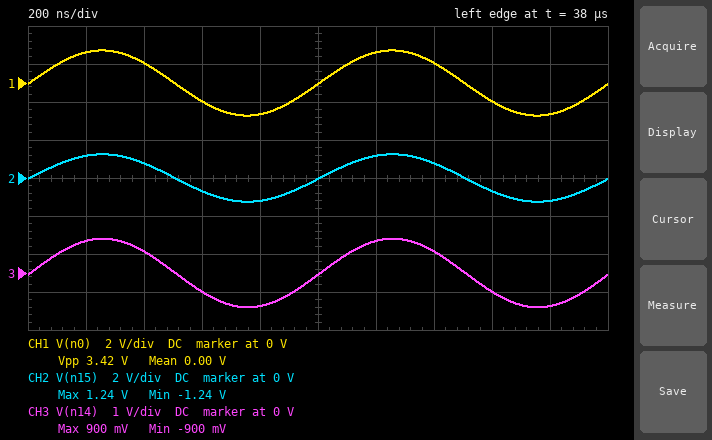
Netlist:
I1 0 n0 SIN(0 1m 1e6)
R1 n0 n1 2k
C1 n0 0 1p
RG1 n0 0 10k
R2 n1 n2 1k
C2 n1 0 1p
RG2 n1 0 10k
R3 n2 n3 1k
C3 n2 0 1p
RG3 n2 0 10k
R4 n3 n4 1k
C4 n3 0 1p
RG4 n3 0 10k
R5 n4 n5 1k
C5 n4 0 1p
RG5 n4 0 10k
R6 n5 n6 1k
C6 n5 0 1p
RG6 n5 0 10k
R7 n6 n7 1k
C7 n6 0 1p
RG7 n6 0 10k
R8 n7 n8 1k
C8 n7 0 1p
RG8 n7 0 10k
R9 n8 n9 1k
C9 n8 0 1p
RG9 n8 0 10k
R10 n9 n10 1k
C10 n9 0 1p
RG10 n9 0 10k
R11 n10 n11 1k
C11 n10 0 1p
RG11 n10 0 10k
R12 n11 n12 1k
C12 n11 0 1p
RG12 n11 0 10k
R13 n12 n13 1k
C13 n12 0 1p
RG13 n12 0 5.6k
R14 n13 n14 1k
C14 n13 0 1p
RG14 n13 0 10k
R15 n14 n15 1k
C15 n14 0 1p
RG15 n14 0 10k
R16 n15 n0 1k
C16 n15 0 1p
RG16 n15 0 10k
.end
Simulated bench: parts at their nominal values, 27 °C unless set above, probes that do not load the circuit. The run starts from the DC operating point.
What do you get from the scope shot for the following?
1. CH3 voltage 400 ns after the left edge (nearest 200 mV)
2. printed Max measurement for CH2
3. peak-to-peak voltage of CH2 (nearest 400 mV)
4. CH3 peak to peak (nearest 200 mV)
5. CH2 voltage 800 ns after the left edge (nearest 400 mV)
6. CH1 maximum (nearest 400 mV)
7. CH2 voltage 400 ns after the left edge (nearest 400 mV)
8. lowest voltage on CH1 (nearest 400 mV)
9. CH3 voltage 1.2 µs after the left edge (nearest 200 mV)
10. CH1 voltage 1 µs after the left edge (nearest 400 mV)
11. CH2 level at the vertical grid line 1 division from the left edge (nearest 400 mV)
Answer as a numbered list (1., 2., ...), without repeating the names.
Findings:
1. 600 mV
2. 1.24 V
3. 2.4 V
4. 1.8 V
5. -1.2 V
6. 1.6 V
7. 800 mV
8. -1.6 V
9. 800 mV
10. 0 V
11. 1.2 V
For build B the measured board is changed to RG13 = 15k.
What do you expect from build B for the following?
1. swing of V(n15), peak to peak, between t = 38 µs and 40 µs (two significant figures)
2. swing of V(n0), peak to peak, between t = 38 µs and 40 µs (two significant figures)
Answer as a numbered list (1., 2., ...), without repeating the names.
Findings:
1. 2.6 V
2. 3.5 V
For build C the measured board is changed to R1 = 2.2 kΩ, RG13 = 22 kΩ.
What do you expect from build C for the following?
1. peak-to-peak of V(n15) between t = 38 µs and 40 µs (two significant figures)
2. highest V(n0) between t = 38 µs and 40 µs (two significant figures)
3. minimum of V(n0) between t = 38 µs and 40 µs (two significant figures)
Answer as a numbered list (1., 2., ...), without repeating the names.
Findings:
1. 2.6 V
2. 1.8 V
3. -1.8 V
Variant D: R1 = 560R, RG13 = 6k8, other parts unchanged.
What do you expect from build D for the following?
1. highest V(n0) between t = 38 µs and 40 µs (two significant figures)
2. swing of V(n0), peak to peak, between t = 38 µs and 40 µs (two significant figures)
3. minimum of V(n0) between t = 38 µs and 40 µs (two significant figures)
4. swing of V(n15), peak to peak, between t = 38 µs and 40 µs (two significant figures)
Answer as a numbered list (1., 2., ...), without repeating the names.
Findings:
1. 1.5 V
2. 3.0 V
3. -1.5 V
4. 2.2 V
